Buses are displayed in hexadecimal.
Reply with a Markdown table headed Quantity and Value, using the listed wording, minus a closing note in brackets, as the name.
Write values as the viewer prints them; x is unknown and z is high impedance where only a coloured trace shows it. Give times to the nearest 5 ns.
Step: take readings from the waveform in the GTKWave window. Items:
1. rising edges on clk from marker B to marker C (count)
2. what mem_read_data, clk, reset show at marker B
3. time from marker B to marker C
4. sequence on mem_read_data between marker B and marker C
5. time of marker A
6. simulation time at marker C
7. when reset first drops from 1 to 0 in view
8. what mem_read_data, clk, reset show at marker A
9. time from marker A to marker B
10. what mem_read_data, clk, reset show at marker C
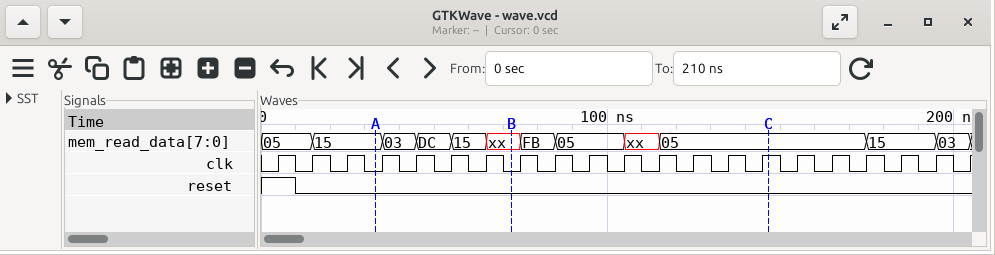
| Quantity | Value |
|---|---|
| rising edges on clk from marker B to marker C | 8 |
| what mem_read_data, clk, reset show at marker B | mem_read_data=xx, clk=0, reset=0 |
| time from marker B to marker C | 75 ns |
| sequence on mem_read_data between marker B and marker C | xx, FB, 05, xx, 05 |
| time of marker A | 35 ns |
| simulation time at marker C | 145 ns |
| when reset first drops from 1 to 0 in view | 10 ns |
| what mem_read_data, clk, reset show at marker A | mem_read_data=15, clk=0, reset=0 |
| time from marker A to marker B | 40 ns |
| what mem_read_data, clk, reset show at marker C | mem_read_data=05, clk=1, reset=0 |
